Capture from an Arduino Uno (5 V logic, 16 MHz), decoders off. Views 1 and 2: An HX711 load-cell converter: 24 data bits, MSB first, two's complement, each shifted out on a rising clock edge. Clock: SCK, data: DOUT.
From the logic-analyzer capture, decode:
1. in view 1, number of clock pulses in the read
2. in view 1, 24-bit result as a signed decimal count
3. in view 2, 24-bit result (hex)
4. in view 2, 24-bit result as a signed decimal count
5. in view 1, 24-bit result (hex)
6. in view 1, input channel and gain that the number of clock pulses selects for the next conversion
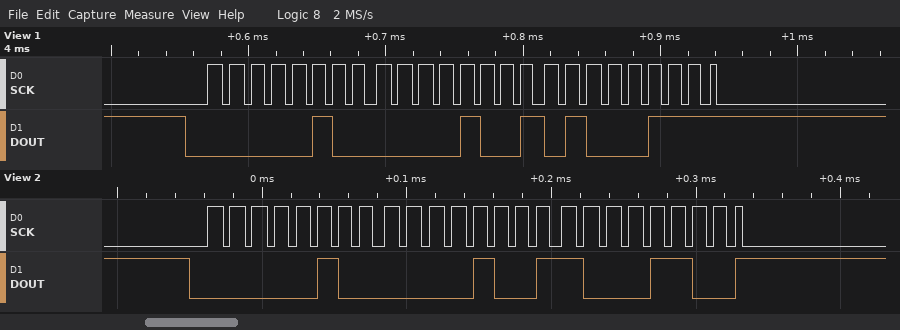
25
264519
0x04098C
264588
0x040947
channel A, gain 128
